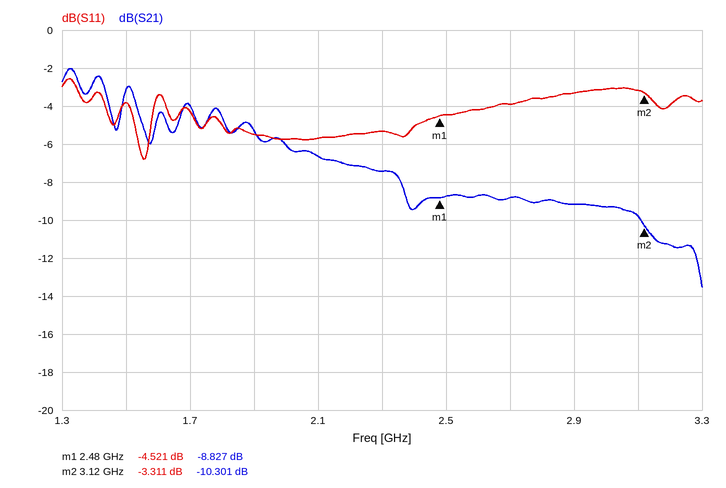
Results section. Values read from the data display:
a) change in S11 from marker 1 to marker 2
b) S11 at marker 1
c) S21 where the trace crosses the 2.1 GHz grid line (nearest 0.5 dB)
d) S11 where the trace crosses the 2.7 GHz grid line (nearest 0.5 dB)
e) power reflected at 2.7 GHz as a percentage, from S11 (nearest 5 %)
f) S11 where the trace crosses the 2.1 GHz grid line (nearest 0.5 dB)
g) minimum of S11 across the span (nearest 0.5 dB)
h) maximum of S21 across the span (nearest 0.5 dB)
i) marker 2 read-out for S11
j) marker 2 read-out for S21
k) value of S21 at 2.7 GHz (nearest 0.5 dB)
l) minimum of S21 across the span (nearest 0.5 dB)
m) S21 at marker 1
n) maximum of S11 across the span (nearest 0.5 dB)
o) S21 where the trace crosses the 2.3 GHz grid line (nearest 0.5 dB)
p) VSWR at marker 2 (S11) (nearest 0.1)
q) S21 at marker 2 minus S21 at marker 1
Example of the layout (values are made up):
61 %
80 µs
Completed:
1.210 dB
-4.521 dB
-6.5 dB
-4.0 dB
40 %
-5.5 dB
-7.0 dB
-2.0 dB
-3.311 dB
-10.301 dB
-9.0 dB
-13.5 dB
-8.827 dB
-2.5 dB
-7.5 dB
5.3
-1.474 dB
